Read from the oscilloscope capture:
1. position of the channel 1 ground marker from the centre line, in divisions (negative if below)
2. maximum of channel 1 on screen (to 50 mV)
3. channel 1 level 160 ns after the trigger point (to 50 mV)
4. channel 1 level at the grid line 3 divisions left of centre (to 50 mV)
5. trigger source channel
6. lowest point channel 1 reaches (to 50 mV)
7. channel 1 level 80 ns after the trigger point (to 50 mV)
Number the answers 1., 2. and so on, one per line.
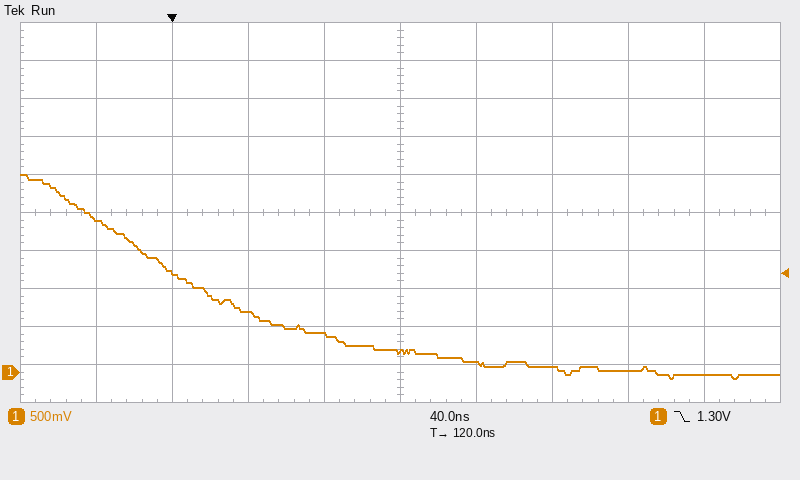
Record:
1. -4.2 div
2. 2.60 V
3. 100 mV
4. 1.30 V
5. channel 1
6. -100 mV
7. 500 mV
